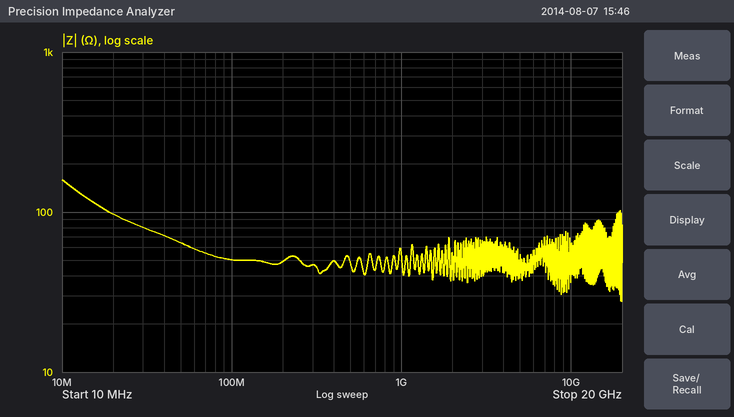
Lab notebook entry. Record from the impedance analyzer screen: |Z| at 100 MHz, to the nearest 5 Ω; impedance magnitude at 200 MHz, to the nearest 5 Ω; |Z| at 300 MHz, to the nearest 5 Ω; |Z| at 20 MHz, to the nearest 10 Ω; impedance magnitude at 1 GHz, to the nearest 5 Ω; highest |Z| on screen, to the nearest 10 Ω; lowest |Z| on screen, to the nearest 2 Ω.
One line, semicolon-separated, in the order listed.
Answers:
50 Ω; 50 Ω; 45 Ω; 100 Ω; 55 Ω; 160 Ω; 28 Ω
